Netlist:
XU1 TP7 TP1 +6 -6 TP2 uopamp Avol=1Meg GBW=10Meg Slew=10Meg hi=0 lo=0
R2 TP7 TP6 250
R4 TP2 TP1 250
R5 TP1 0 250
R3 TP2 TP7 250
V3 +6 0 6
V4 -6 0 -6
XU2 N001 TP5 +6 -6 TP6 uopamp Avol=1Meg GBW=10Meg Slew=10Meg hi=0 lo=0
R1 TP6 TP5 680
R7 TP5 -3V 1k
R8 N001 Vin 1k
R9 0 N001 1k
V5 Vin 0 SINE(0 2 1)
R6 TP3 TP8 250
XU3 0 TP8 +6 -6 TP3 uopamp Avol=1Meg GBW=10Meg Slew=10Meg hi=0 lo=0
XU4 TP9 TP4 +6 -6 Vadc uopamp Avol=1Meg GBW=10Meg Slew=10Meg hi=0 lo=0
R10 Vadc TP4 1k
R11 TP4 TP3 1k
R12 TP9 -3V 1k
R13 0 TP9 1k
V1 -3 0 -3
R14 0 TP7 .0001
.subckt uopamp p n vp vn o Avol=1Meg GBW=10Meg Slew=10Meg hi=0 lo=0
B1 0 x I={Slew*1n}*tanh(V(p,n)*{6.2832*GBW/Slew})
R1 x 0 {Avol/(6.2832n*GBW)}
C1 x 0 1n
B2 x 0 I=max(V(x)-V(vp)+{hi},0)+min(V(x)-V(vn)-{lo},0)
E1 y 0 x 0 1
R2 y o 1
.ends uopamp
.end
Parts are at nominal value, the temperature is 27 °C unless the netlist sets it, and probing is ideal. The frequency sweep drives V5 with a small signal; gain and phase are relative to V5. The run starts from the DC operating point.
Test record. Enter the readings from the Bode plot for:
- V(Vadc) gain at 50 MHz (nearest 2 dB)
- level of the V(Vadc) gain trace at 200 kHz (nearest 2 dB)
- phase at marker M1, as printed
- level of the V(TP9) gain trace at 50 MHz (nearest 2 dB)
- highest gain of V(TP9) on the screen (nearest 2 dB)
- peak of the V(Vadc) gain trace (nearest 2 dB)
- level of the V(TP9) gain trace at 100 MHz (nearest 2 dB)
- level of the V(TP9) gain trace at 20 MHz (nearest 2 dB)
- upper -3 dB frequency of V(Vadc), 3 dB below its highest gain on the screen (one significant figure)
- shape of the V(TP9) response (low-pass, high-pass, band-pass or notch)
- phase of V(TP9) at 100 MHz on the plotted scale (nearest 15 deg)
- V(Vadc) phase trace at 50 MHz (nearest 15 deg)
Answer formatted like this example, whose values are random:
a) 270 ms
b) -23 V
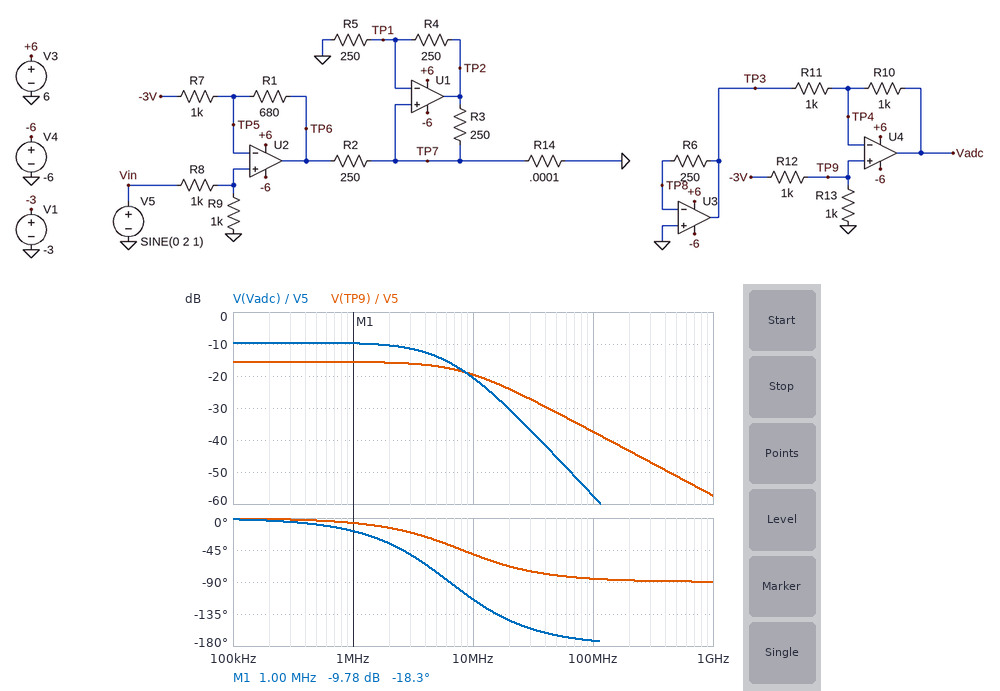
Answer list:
a) -46 dB
b) -10 dB
c) -18.3 deg
d) -32 dB
e) -16 dB
f) -10 dB
g) -38 dB
h) -24 dB
i) 4 MHz
j) low-pass
k) -90 deg
l) -165 deg
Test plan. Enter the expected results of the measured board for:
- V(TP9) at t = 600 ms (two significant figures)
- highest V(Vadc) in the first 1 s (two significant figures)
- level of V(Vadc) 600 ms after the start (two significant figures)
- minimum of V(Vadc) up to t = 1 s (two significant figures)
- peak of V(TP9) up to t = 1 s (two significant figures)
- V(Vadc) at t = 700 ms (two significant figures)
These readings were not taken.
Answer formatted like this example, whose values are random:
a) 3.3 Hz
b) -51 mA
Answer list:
a) -200 mV
b) 670 mV
c) -390 mV
d) -670 mV
e) 330 mV
f) -630 mV
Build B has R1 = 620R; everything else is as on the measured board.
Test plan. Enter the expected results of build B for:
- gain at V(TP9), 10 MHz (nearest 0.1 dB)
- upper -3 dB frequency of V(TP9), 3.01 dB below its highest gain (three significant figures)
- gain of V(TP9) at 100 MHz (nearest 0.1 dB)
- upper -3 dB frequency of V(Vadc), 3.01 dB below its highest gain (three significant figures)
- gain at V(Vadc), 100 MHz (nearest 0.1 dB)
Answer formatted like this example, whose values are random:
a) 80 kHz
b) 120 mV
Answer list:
a) -19.5 dB
b) 8.25 MHz
c) -37.3 dB
d) 3.95 MHz
e) -57.3 dB
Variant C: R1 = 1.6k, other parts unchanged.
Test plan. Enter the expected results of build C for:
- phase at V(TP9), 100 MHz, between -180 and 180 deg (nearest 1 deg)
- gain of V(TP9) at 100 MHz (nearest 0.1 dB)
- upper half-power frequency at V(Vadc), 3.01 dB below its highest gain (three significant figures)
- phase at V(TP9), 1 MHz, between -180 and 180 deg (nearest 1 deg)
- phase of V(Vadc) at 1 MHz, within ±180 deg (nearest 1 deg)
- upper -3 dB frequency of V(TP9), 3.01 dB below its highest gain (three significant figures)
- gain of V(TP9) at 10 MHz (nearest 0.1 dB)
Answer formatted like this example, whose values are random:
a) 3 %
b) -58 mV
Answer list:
a) -86 deg
b) -39.3 dB
c) 3.62 MHz
d) -9 deg
e) -20 deg
f) 6.49 MHz
g) -20.8 dB
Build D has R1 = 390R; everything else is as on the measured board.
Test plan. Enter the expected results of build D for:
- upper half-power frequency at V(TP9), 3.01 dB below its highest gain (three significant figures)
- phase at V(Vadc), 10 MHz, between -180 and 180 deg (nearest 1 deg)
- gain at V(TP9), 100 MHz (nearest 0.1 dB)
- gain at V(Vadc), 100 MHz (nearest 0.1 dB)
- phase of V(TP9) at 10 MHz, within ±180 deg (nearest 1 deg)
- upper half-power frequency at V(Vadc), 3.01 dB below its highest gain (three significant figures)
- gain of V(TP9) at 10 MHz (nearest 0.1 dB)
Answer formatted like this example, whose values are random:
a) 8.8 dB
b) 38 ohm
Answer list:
a) 8.81 MHz
b) -112 deg
c) -36.7 dB
d) -56.7 dB
e) -49 deg
f) 4.04 MHz
g) -19.2 dB
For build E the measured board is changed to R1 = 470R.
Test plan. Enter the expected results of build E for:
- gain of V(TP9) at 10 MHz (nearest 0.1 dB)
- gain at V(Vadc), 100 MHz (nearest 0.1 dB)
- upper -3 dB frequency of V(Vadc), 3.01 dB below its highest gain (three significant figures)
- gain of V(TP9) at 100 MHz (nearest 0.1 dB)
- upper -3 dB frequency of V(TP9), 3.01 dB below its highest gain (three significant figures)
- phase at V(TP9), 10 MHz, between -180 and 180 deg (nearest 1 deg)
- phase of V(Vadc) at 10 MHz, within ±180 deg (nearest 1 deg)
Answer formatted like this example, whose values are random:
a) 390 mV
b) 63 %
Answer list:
a) -19.3 dB
b) -56.9 dB
c) 4.01 MHz
d) -36.9 dB
e) 8.61 MHz
f) -49 deg
g) -113 deg
